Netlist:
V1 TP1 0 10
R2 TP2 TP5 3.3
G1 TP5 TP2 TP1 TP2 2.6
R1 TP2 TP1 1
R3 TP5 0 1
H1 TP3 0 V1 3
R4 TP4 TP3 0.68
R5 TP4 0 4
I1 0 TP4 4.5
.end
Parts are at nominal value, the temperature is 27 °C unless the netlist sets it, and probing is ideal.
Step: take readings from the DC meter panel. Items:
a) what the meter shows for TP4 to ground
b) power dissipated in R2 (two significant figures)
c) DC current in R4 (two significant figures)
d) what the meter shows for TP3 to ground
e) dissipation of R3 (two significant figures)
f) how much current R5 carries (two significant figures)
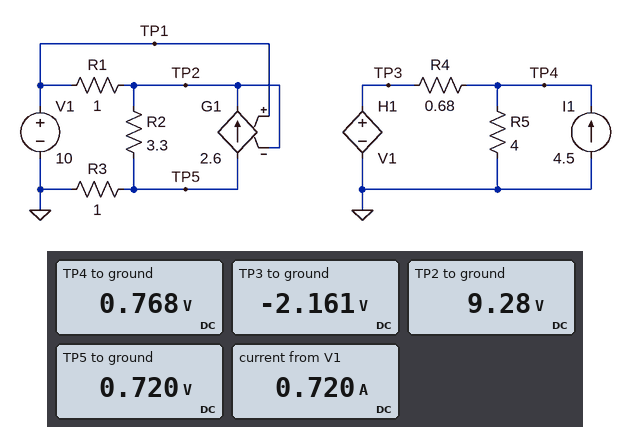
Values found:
0.768 V
22 W
4.3 A
-2.161 V
520 mW
190 mA
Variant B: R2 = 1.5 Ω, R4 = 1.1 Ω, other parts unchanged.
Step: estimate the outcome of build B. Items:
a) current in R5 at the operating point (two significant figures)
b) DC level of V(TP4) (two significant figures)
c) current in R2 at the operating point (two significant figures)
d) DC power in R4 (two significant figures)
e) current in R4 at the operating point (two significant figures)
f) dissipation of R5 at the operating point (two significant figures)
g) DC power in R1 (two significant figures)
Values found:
180 mA
700 mV
4.9 A
21 W
4.3 A
120 mW
1.8 W
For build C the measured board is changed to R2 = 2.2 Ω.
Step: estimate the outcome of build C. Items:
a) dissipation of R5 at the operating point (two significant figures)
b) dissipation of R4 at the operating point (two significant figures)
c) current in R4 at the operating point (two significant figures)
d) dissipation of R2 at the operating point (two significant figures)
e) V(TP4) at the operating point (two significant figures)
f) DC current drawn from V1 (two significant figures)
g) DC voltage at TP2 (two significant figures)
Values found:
230 µW
14 W
4.5 A
29 W
31 mV
1.0 A
9.0 V
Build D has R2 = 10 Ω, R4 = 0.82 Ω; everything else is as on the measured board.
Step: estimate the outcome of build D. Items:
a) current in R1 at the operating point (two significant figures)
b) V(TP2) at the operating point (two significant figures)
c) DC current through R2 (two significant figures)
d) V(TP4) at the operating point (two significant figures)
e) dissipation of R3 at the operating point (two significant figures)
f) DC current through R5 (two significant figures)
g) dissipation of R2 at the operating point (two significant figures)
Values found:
260 mA
9.7 V
950 mA
2.4 V
69 mW
600 mA
9.0 W
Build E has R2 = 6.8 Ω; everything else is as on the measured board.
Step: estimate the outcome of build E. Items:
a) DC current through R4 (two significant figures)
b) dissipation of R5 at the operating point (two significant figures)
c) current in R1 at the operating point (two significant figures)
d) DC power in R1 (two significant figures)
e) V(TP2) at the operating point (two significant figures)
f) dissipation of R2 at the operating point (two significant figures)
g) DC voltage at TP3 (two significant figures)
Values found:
4.1 A
680 mW
380 mA
140 mW
9.6 V
13 W
-1.1 V
